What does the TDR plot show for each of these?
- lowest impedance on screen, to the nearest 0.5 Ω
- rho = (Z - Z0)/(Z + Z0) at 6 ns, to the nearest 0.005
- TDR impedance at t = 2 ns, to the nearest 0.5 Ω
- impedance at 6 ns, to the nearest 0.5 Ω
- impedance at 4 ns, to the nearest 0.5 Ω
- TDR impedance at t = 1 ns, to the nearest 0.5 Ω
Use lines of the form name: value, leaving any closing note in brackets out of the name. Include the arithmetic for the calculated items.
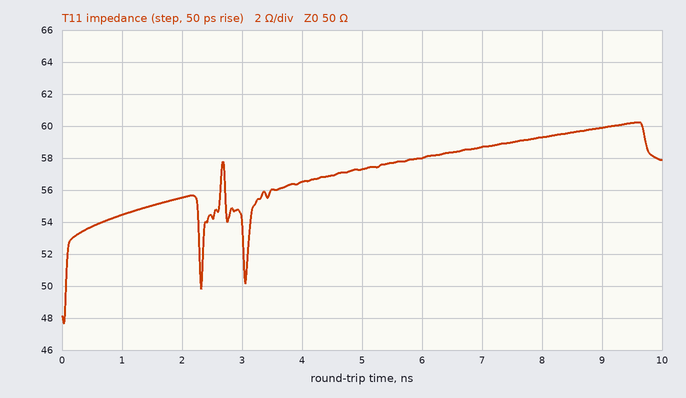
lowest impedance on screen, to the nearest 0.5 Ω: 47.5 Ω
rho = (Z - Z0)/(Z + Z0) at 6 ns, to the nearest 0.005: (58 − 50)/(58 + 50) ≈ +0.0741, so +0.075 to the nearest 0.005
TDR impedance at t = 2 ns, to the nearest 0.5 Ω: 55.5 Ω
impedance at 6 ns, to the nearest 0.5 Ω: 58.0 Ω
impedance at 4 ns, to the nearest 0.5 Ω: 56.5 Ω
TDR impedance at t = 1 ns, to the nearest 0.5 Ω: 54.5 Ω
